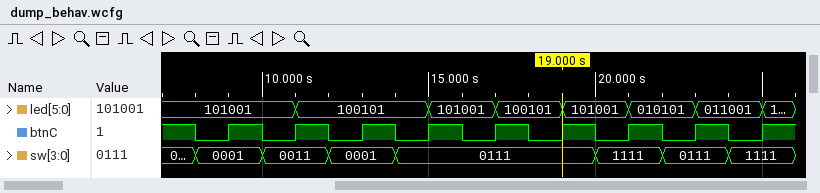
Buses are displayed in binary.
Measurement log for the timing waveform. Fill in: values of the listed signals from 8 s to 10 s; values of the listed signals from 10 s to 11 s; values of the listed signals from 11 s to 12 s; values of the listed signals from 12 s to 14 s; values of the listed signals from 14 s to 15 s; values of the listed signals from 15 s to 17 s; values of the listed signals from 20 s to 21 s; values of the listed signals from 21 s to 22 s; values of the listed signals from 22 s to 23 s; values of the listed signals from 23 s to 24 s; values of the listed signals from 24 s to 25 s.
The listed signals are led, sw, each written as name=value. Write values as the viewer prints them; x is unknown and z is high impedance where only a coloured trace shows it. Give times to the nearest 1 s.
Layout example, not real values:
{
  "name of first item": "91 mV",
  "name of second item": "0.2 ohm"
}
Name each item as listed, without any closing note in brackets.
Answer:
{
  "values of the listed signals from 8 s to 10 s": "led=101001, sw=0001",
  "values of the listed signals from 10 s to 11 s": "led=101001, sw=0011",
  "values of the listed signals from 11 s to 12 s": "led=100101, sw=0011",
  "values of the listed signals from 12 s to 14 s": "led=100101, sw=0001",
  "values of the listed signals from 14 s to 15 s": "led=100101, sw=0111",
  "values of the listed signals from 15 s to 17 s": "led=101001, sw=0111",
  "values of the listed signals from 20 s to 21 s": "led=101001, sw=1111",
  "values of the listed signals from 21 s to 22 s": "led=010101, sw=1111",
  "values of the listed signals from 22 s to 23 s": "led=010101, sw=0111",
  "values of the listed signals from 23 s to 24 s": "led=011001, sw=0111",
  "values of the listed signals from 24 s to 25 s": "led=011001, sw=1111"
}
